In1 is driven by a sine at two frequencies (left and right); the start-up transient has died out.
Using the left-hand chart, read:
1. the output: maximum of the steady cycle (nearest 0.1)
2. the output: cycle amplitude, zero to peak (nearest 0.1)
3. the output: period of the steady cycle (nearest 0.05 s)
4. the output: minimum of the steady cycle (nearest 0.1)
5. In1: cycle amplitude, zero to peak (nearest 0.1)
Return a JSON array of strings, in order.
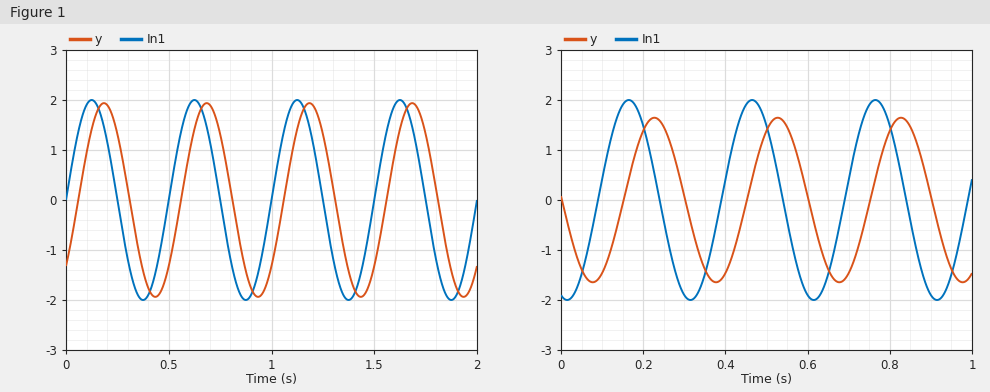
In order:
["1.9", "1.9", "0.50 s", "-1.9", "2.0"]
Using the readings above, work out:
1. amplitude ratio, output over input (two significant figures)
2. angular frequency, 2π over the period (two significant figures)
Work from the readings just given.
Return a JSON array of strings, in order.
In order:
["0.95", "13 rad/s"]
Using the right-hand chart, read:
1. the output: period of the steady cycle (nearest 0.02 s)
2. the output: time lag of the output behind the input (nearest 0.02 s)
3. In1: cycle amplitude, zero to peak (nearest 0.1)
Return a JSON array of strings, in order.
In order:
["0.30 s", "0.06 s", "2.0"]
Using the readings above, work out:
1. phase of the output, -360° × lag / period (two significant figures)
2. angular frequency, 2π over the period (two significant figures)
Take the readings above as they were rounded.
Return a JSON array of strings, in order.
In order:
["-72°", "21 rad/s"]
